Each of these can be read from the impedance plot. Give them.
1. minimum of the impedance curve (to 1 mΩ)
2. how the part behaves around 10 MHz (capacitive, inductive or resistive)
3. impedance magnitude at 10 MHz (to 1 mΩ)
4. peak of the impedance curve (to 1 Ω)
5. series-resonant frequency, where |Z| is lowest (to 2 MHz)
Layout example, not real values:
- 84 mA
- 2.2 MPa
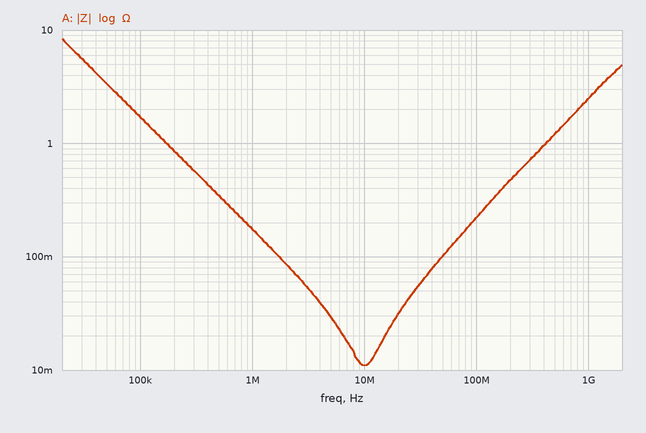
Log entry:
- 11 mΩ
- resistive
- 11 mΩ
- 8 Ω
- 10 MHz
